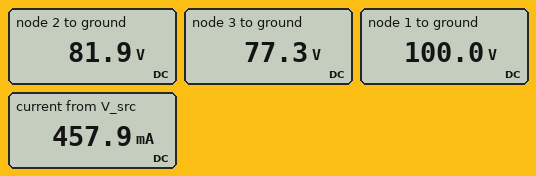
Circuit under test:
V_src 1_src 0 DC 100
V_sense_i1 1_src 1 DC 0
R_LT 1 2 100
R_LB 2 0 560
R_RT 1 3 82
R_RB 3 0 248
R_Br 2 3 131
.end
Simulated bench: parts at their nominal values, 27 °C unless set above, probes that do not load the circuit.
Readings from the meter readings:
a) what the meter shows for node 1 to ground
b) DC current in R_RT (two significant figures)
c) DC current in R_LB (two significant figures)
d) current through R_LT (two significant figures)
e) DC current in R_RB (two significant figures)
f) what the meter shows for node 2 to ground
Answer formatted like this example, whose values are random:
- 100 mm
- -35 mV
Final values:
- 100.0 V
- 280 mA
- 150 mA
- 180 mA
- 310 mA
- 81.9 V
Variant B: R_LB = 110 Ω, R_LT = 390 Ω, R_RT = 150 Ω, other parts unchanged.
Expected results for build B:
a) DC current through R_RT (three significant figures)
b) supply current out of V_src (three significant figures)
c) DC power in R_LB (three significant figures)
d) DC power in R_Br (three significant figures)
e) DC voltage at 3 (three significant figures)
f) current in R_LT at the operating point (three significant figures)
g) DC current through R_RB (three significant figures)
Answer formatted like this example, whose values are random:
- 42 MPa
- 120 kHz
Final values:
- 332 mA
- 504 mA
- 9.99 W
- 2.21 W
- 50.2 V
- 171 mA
- 202 mA
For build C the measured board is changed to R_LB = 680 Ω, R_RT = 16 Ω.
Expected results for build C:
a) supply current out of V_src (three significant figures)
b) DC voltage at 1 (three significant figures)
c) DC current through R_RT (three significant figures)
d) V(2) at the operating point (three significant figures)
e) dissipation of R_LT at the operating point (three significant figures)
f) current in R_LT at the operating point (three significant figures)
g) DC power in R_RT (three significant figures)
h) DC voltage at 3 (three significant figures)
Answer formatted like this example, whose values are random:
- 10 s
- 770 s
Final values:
- 509 mA
- 100 V
- 406 mA
- 89.7 V
- 1.06 W
- 103 mA
- 2.64 W
- 93.5 V
